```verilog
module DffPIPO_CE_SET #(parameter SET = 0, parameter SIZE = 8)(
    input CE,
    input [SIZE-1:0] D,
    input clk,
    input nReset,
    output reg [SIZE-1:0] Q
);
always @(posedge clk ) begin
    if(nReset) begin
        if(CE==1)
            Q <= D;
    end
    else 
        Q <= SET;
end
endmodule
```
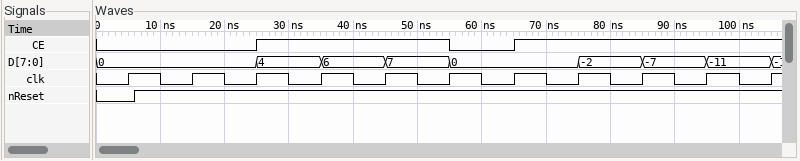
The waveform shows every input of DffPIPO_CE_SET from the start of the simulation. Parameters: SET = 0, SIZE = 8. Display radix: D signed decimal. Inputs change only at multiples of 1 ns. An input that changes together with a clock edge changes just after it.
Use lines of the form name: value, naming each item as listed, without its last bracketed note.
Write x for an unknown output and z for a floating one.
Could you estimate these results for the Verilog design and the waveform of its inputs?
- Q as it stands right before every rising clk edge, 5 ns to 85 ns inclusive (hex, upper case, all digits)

Q as it stands right before every rising clk edge, 5 ns to 85 ns inclusive: x, 00, 00, 00, 04, 06, 07, 07, 00
